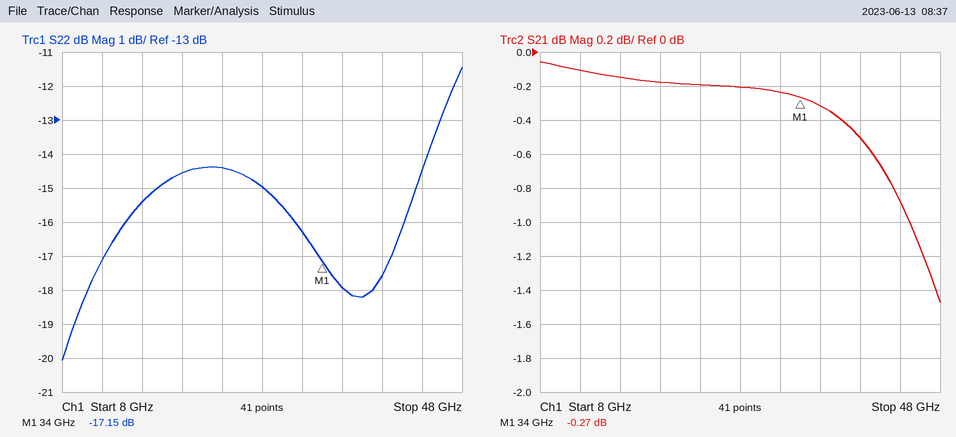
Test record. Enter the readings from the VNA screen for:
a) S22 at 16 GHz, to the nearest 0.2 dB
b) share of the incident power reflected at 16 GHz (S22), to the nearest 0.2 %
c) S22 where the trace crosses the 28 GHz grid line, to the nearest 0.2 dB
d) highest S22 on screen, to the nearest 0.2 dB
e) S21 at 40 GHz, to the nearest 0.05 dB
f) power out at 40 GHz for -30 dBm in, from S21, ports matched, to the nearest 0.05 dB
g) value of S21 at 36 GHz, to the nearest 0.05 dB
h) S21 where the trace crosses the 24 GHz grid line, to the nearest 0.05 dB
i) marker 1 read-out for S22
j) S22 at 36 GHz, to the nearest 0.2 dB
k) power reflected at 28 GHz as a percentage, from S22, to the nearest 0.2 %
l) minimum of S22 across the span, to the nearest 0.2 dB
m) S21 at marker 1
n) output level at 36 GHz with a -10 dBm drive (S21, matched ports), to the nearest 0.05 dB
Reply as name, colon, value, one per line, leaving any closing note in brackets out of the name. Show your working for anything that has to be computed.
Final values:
S22 at 16 GHz, to the nearest 0.2 dB: -15.4 dB
share of the incident power reflected at 16 GHz (S22), to the nearest 0.2 %: 10^(-15.4/10) ≈ 2.88 %, so 2.8 % to the nearest 0.2 %
S22 where the trace crosses the 28 GHz grid line, to the nearest 0.2 dB: -15.0 dB
highest S22 on screen, to the nearest 0.2 dB: -11.4 dB
S21 at 40 GHz, to the nearest 0.05 dB: -0.50 dB
power out at 40 GHz for -30 dBm in, from S21, ports matched, to the nearest 0.05 dB: -30 dBm + (-0.50 dB) = -30.50 dBm
value of S21 at 36 GHz, to the nearest 0.05 dB: -0.30 dB
S21 where the trace crosses the 24 GHz grid line, to the nearest 0.05 dB: -0.20 dB
marker 1 read-out for S22: -17.15 dB
S22 at 36 GHz, to the nearest 0.2 dB: -18.0 dB
power reflected at 28 GHz as a percentage, from S22, to the nearest 0.2 %: 10^(-15/10) ≈ 3.2 %
minimum of S22 across the span, to the nearest 0.2 dB: -20.0 dB
S21 at marker 1: -0.27 dB
output level at 36 GHz with a -10 dBm drive (S21, matched ports), to the nearest 0.05 dB: -10 dBm + (-0.30 dB) = -10.30 dBm
